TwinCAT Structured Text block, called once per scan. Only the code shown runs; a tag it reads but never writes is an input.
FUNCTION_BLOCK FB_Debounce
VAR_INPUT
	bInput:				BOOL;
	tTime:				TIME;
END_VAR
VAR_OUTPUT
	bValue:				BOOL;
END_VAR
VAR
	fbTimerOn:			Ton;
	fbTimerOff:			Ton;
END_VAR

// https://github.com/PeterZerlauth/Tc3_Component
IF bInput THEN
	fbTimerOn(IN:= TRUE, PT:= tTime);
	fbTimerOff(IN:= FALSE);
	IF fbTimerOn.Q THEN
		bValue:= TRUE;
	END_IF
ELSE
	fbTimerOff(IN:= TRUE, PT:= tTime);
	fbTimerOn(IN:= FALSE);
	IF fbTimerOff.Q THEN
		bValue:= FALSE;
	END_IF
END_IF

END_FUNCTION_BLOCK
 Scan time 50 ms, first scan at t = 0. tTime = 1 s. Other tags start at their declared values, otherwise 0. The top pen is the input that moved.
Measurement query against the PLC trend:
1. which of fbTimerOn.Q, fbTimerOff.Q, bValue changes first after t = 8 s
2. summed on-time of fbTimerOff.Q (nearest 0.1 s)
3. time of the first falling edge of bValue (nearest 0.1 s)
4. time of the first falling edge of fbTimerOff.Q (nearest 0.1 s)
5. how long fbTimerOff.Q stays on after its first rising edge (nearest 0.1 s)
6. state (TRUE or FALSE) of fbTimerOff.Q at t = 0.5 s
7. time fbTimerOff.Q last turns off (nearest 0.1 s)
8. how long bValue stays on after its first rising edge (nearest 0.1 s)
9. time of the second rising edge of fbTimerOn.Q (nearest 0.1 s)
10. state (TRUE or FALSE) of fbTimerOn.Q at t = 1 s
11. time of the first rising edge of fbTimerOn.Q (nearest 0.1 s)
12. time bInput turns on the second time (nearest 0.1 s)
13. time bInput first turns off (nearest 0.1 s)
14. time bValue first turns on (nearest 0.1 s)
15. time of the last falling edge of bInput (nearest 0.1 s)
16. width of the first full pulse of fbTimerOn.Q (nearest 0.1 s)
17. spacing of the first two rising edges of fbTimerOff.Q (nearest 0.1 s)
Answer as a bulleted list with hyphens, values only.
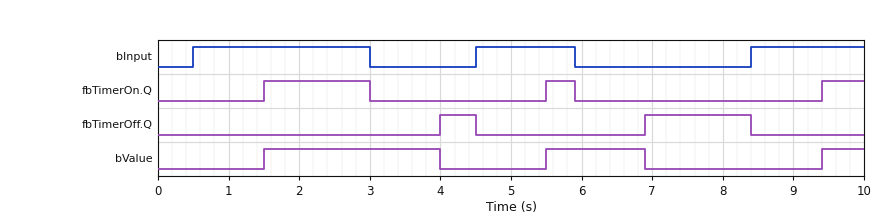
- fbTimerOff.Q
- 2.0 s
- 4.0 s
- 4.5 s
- 0.5 s
- FALSE
- 8.4 s
- 2.5 s
- 5.5 s
- FALSE
- 1.5 s
- 4.5 s
- 3.0 s
- 1.5 s
- 5.9 s
- 1.5 s
- 2.9 s
